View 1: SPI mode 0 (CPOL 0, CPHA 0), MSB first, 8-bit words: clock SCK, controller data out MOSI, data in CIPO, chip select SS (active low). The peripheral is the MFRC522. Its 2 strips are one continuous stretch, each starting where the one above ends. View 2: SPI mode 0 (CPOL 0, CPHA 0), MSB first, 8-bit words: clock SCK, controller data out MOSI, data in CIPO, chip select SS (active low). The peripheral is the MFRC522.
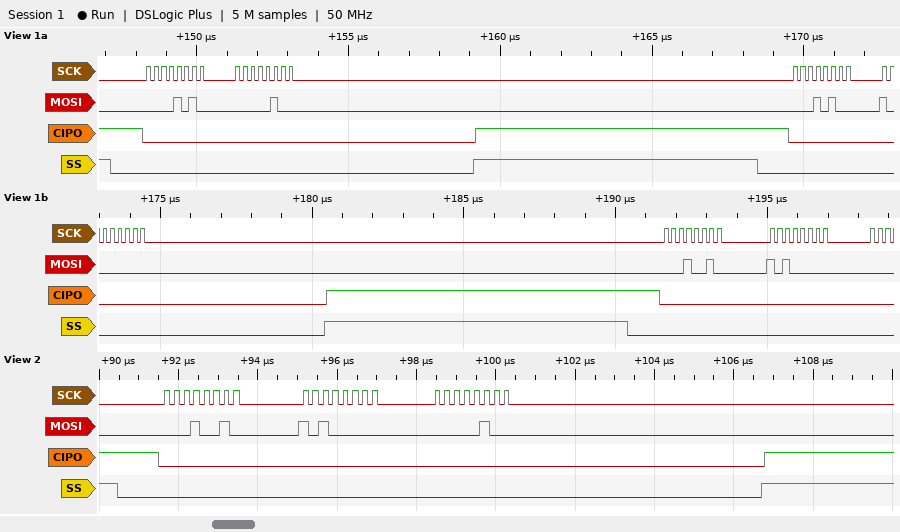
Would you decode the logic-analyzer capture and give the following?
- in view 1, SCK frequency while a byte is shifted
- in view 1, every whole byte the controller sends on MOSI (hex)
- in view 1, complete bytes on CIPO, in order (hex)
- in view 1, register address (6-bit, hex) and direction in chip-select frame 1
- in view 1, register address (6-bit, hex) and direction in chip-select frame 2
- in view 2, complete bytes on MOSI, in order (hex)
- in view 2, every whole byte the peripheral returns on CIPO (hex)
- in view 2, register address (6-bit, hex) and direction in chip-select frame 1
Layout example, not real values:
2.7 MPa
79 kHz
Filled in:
4 MHz
0A 04 14 80 12 A0
00 00 00 00 00 00
0x05 write
0x0A write
0x12 0xA0 0x04
0x00 0x00 0x00
0x09 write
